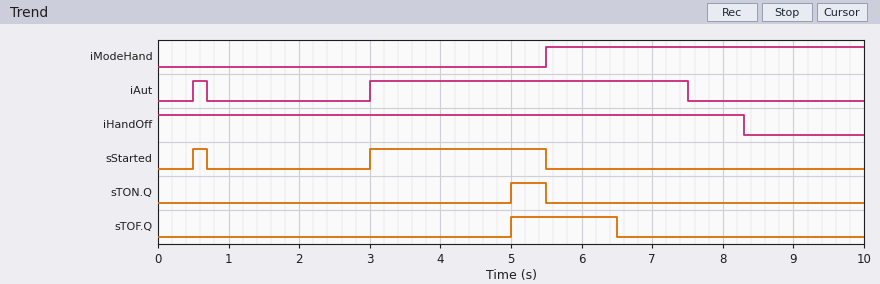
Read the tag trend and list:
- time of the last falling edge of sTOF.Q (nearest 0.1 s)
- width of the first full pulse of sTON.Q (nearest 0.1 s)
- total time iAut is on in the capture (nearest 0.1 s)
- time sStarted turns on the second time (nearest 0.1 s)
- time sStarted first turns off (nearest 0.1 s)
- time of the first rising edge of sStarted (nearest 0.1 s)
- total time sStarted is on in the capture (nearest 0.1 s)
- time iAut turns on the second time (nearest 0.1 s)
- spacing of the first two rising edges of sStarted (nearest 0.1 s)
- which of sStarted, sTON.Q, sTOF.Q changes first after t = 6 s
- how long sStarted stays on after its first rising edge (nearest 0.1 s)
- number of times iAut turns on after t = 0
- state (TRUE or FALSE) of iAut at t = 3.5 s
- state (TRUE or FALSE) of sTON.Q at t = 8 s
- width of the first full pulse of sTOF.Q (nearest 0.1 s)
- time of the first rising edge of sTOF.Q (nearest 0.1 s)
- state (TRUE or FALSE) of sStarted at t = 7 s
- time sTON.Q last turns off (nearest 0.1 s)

6.5 s
0.5 s
4.7 s
3.0 s
0.7 s
0.5 s
2.7 s
3.0 s
2.5 s
sTOF.Q
0.2 s
2
TRUE
FALSE
1.5 s
5.0 s
FALSE
5.5 s
